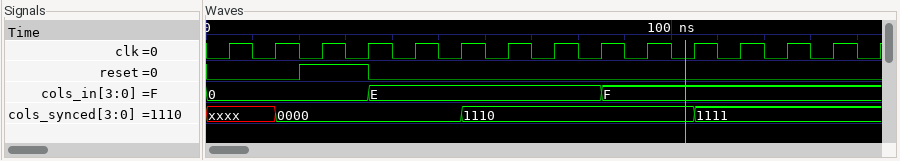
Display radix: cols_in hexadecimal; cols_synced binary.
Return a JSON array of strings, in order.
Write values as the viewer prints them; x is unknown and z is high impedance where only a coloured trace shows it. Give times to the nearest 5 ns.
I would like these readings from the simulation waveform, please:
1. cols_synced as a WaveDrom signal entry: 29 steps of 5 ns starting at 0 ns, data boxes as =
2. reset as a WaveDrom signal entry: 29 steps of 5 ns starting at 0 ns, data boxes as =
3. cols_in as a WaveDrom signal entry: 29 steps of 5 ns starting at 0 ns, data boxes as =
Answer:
["{name: 'cols_synced', wave: 'x..=.......=.........=.......', data: '0000 1110 1111'}", "{name: 'reset', wave: '0...1..0.....................'}", "{name: 'cols_in', wave: '=......=.........=...........', data: '0 E F'}"]
